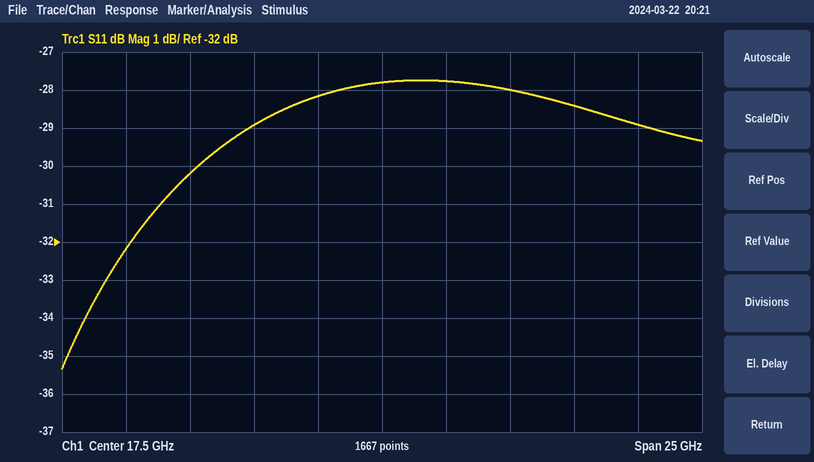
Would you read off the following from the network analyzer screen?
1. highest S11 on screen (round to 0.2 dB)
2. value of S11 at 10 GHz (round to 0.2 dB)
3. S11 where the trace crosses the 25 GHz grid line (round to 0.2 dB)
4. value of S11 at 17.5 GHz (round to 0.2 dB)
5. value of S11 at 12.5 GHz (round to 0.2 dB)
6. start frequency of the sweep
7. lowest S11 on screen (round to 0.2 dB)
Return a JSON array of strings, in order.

["-27.8 dB", "-30.2 dB", "-28.4 dB", "-27.8 dB", "-29.0 dB", "5 GHz", "-35.4 dB"]
